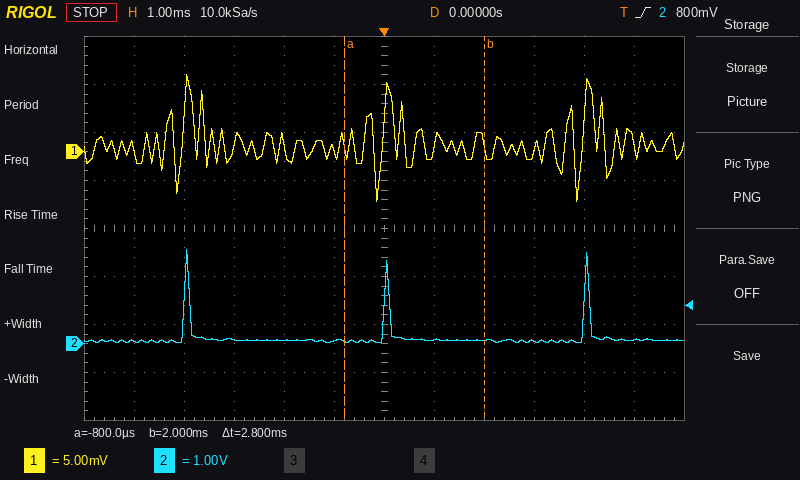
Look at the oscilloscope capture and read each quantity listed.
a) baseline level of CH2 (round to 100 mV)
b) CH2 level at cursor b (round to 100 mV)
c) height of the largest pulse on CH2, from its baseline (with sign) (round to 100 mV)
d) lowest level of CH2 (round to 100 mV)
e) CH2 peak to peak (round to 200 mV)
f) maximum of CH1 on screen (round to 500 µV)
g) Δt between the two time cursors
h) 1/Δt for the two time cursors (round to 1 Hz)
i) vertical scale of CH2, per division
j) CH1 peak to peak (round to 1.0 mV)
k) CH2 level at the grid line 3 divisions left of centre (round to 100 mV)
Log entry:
100 mV
100 mV
+1.9 V
0.0 V
2.0 V
8.0 mV
2.8 ms
357 Hz
1 V
13.0 mV
100 mV
